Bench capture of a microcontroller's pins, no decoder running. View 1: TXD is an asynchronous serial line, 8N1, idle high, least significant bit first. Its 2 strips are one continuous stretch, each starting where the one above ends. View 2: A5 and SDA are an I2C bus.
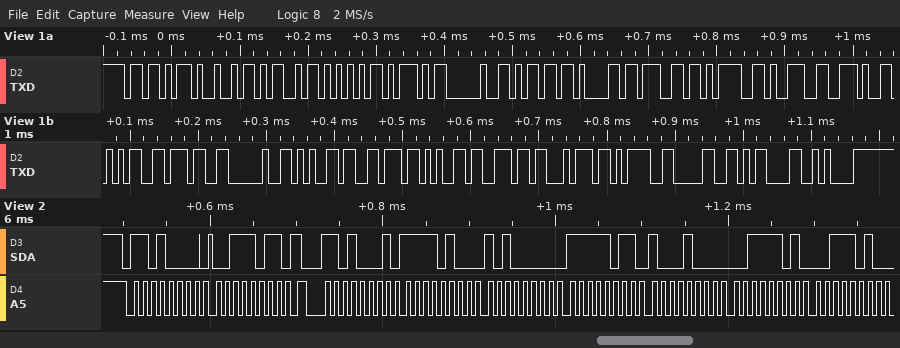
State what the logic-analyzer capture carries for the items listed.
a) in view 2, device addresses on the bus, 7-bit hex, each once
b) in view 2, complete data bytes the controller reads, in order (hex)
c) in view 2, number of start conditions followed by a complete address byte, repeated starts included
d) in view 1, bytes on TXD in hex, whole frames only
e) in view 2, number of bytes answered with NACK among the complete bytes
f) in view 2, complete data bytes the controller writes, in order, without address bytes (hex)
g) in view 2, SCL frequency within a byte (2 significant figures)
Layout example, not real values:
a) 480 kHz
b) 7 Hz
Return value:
a) 0x68
b) F4 A0 FB 88 3D 3A
c) 2
d) 0x5B 0x49 0x4D 0x55 0x5D 0x20 0x6D 0x61 0x67 0x3D 0x39 0x2E 0x35 0x37 0x20 0x65 0x76 0x65 0x6E 0x74 0x3D 0x30 0x0D 0x0A
e) 0
f) 3B
g) 100 kHz
